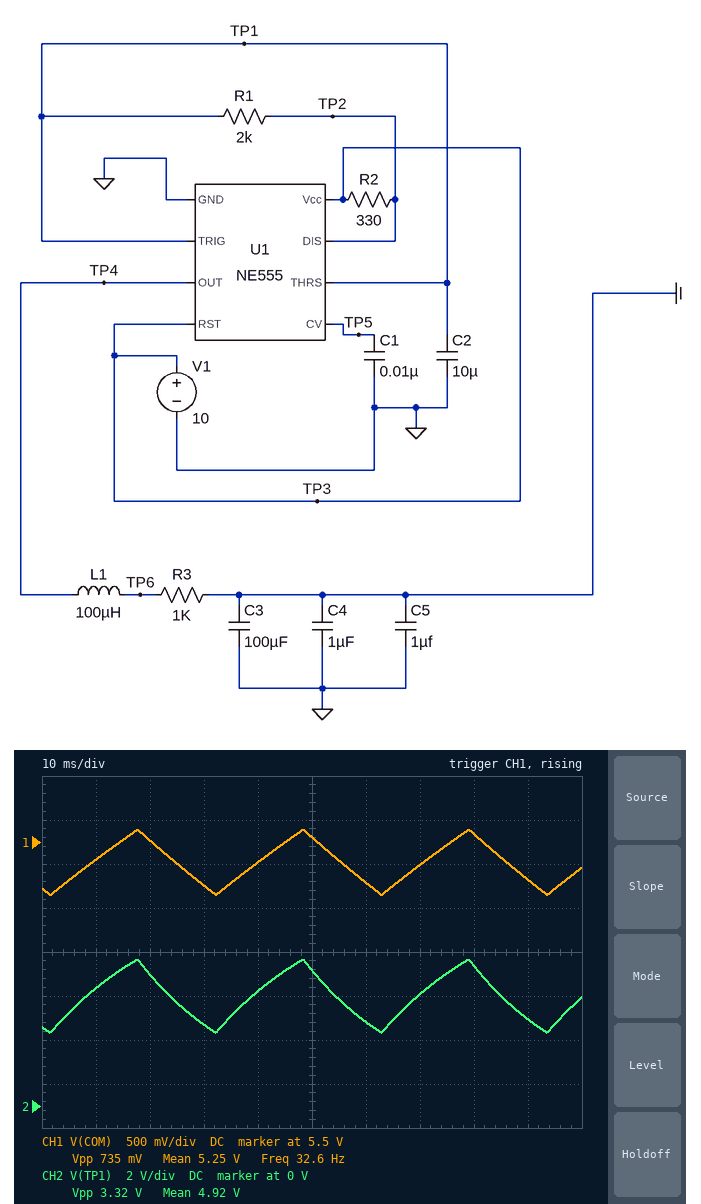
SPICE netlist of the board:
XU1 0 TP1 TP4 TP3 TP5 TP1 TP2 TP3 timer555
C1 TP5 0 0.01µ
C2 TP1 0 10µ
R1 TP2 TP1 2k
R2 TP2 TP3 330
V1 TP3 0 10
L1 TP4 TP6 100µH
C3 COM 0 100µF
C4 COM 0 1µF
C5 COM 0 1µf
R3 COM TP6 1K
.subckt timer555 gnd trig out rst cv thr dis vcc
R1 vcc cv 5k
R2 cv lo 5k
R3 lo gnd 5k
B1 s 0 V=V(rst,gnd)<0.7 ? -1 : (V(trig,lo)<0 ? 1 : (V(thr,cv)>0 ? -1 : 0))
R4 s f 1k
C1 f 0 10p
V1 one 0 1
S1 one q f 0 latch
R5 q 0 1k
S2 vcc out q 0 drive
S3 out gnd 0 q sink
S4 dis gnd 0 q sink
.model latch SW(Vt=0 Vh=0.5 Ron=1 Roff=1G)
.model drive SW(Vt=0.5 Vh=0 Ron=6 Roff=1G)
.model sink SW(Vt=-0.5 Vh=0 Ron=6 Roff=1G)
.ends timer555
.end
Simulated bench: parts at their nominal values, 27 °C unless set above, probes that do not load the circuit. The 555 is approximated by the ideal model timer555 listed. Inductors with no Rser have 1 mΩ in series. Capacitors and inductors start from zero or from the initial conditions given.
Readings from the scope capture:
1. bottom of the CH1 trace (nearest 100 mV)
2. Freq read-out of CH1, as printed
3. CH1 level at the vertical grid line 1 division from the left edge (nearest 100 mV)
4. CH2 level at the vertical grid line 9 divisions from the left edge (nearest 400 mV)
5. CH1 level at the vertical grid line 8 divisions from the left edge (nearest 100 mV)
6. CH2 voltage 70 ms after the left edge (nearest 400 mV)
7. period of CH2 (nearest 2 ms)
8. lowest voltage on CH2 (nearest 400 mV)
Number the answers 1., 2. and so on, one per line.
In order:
1. 4.9 V
2. 32.6 Hz
3. 5.3 V
4. 4.0 V
5. 5.6 V
6. 5.2 V
7. 30 ms
8. 3.2 V
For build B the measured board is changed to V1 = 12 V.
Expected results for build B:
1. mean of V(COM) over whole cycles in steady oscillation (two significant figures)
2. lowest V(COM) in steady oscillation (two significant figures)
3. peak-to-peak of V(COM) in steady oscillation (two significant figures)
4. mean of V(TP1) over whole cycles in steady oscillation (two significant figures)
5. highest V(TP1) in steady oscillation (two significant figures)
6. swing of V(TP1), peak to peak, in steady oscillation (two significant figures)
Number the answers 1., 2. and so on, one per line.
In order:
1. 6.3 V
2. 5.9 V
3. 890 mV
4. 6.0 V
5. 8.0 V
6. 4.0 V
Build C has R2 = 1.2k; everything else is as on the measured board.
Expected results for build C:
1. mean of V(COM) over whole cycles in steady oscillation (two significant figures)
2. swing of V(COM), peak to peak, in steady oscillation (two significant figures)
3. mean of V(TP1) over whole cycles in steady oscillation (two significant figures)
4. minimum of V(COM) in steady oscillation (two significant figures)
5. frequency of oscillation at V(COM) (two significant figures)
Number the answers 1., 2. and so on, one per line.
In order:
1. 6.1 V
2. 840 mV
3. 5.0 V
4. 5.7 V
5. 28 Hz
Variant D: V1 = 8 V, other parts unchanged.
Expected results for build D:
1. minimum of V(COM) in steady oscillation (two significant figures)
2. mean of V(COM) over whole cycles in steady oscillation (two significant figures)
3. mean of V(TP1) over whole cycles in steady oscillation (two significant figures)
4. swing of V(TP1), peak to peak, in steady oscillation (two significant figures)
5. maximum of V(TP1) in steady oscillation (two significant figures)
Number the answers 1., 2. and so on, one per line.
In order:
1. 3.9 V
2. 4.2 V
3. 4.0 V
4. 2.7 V
5. 5.3 V
